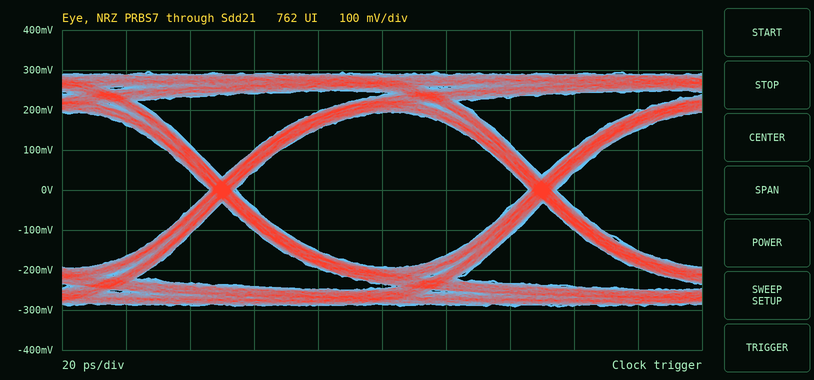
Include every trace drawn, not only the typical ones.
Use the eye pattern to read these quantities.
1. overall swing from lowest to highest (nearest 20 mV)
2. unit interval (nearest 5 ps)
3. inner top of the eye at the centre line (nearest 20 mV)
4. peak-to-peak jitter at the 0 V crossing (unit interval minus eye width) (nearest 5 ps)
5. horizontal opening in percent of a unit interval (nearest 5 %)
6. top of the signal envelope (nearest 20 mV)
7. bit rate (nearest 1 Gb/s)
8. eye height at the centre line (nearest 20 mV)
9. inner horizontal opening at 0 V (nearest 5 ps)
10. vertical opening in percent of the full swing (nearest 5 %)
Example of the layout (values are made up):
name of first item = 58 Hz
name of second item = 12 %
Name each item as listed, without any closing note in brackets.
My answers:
overall swing from lowest to highest = 580 mV
unit interval = 100 ps
inner top of the eye at the centre line = 200 mV
peak-to-peak jitter at the 0 V crossing (unit interval minus eye width) = 10 ps
horizontal opening in percent of a unit interval = 90 %
top of the signal envelope = 300 mV
bit rate = 10 Gb/s
eye height at the centre line = 380 mV
inner horizontal opening at 0 V = 90 ps
vertical opening in percent of the full swing = 65 %
